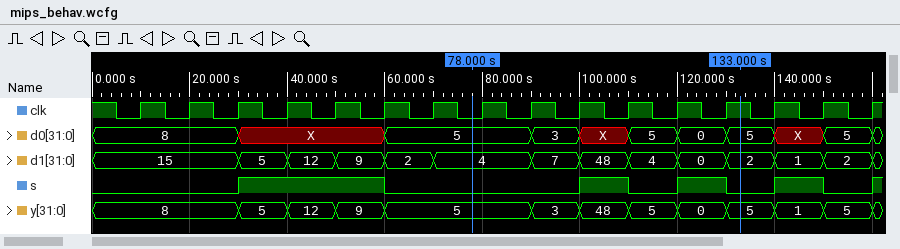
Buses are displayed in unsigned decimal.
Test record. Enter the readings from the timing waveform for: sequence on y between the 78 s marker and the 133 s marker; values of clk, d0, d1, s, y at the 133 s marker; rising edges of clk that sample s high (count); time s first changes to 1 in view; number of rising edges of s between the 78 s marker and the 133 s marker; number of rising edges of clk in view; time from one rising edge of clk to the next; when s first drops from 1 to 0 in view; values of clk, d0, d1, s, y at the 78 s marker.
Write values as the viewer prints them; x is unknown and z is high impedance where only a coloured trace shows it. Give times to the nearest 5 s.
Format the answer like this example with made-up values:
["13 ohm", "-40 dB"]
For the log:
["5, 3, 48, 5, 0, 5", "clk=1, d0=5, d1=2, s=0, y=5", "6", "30 s", "2", "16", "10 s", "60 s", "clk=0, d0=5, d1=4, s=0, y=5"]
